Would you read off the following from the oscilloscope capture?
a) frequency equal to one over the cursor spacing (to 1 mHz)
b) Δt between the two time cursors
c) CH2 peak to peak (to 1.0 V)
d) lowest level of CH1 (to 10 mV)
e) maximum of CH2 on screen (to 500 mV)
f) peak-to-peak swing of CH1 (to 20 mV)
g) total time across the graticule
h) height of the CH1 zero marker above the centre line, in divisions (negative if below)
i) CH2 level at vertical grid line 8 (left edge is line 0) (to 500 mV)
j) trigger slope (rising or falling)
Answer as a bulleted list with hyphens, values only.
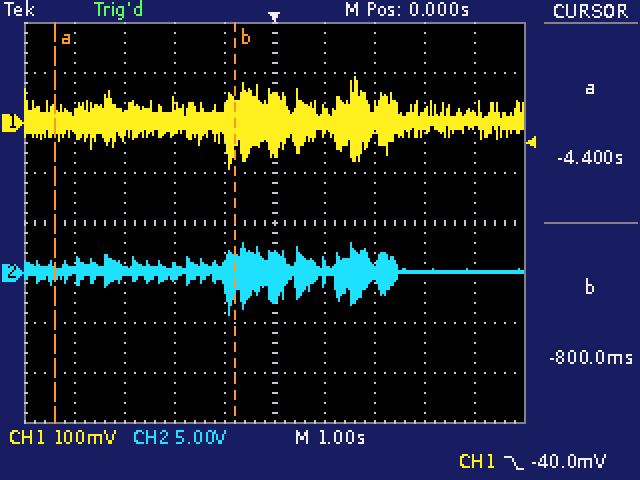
- 278 mHz
- 3.6 s
- 7.0 V
- -90 mV
- 3.0 V
- 180 mV
- 10 s
- +2.0 div
- 0.0 V
- falling
